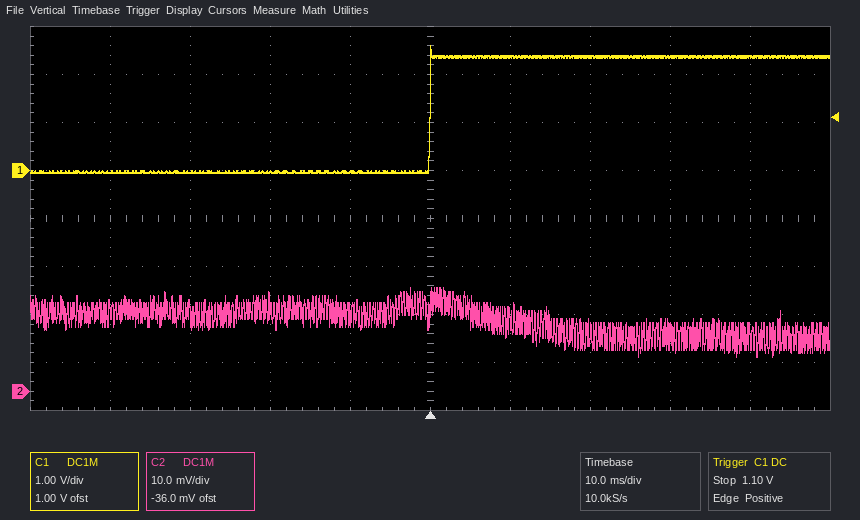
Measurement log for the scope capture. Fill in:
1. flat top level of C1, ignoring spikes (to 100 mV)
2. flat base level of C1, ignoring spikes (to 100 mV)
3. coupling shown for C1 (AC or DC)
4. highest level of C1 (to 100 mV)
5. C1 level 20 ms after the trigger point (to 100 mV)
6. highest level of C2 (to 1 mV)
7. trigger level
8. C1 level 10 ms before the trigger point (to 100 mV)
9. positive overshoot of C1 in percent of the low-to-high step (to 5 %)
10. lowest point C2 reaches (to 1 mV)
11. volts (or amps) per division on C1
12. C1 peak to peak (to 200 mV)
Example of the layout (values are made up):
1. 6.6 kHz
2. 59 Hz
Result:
1. 2.4 V
2. 0.0 V
3. DC
4. 2.6 V
5. 2.4 V
6. 22 mV
7. 1.10 V
8. 0.0 V
9. 10 %
10. 7 mV
11. 1 V
12. 2.6 V
